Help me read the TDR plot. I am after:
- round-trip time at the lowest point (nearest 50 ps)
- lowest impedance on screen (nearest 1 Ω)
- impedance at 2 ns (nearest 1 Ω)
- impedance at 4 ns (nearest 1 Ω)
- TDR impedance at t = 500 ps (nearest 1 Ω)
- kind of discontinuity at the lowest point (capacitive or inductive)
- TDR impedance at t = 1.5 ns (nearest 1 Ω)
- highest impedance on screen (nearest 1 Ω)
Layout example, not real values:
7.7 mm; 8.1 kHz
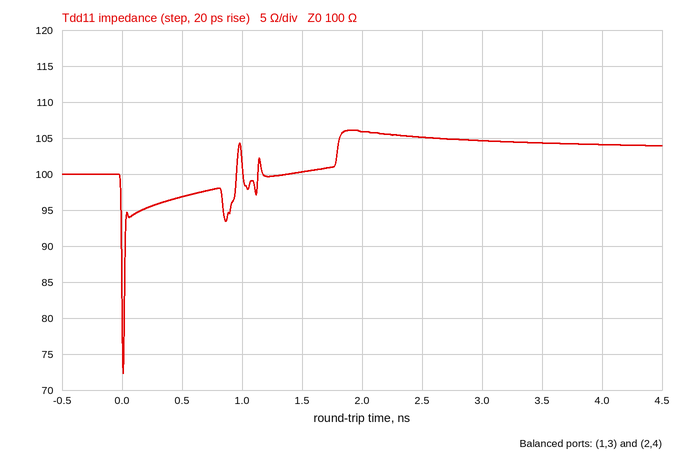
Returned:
0 ps; 72 Ω; 106 Ω; 104 Ω; 97 Ω; capacitive; 100 Ω; 106 Ω
